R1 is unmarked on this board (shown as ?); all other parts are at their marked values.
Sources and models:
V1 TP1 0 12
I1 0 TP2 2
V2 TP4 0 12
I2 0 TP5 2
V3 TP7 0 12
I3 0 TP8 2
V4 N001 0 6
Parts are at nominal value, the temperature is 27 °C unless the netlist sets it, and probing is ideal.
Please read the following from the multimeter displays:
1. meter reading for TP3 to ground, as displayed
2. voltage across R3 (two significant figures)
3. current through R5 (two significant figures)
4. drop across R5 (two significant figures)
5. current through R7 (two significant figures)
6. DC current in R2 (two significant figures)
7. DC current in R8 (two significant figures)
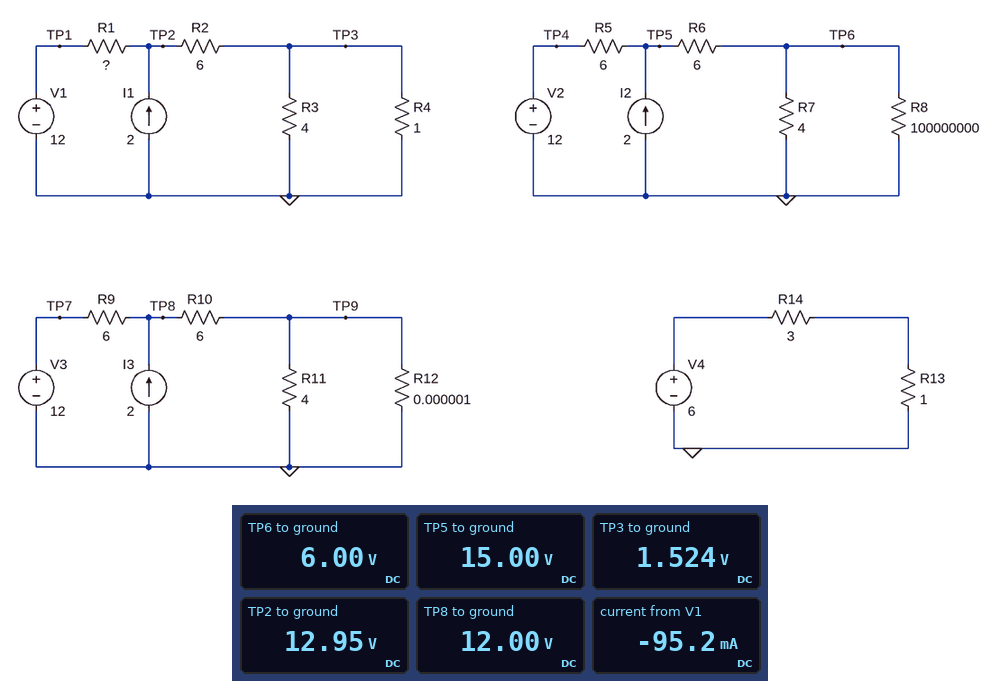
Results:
1.524 V
1.5 V
500 mA
3.0 V
1.5 A
1.9 A
60 nA
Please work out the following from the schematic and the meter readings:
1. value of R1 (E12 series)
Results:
10 Ω
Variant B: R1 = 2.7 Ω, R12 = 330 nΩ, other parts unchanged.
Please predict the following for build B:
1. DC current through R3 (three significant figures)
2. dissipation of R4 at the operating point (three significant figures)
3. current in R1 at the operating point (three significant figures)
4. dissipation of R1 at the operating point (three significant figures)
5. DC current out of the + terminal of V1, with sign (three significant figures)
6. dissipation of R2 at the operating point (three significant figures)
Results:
366 mA
2.15 W
168 mA
76.6 mW
-168 mA
20.1 W
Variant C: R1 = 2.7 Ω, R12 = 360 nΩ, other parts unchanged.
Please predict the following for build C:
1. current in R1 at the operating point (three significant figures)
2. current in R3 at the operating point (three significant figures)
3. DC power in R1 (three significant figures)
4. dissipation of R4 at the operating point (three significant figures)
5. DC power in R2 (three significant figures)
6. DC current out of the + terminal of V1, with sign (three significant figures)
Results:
168 mA
366 mA
76.6 mW
2.15 W
20.1 W
-168 mA
